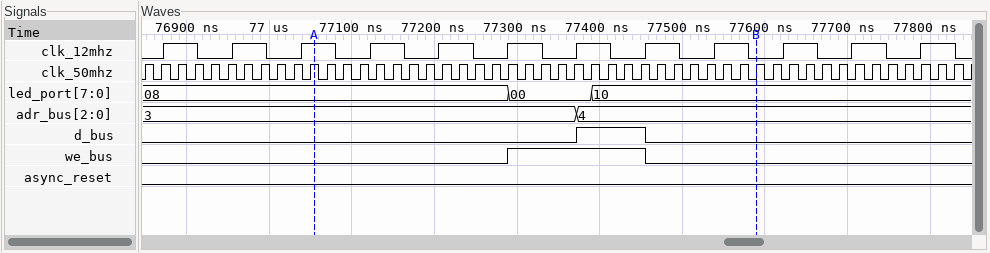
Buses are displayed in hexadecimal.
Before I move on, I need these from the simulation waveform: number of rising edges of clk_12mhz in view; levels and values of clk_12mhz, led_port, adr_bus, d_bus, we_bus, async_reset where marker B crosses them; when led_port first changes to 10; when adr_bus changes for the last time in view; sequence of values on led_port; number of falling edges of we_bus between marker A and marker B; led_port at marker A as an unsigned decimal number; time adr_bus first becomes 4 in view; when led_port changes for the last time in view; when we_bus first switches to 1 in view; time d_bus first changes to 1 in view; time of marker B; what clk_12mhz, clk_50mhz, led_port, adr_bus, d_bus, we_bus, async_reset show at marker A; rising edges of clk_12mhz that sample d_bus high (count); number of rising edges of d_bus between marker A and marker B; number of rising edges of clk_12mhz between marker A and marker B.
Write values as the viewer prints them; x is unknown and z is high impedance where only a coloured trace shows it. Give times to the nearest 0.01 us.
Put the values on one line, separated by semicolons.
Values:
12; clk_12mhz=0, led_port=10, adr_bus=4, d_bus=0, we_bus=0, async_reset=0; 77.39 us; 77.37 us; 08, 00, 10; 1; 8; 77.37 us; 77.39 us; 77.29 us; 77.37 us; 77.59 us; clk_12mhz=1, clk_50mhz=1, led_port=08, adr_bus=3, d_bus=0, we_bus=0, async_reset=0; 1; 1; 6
